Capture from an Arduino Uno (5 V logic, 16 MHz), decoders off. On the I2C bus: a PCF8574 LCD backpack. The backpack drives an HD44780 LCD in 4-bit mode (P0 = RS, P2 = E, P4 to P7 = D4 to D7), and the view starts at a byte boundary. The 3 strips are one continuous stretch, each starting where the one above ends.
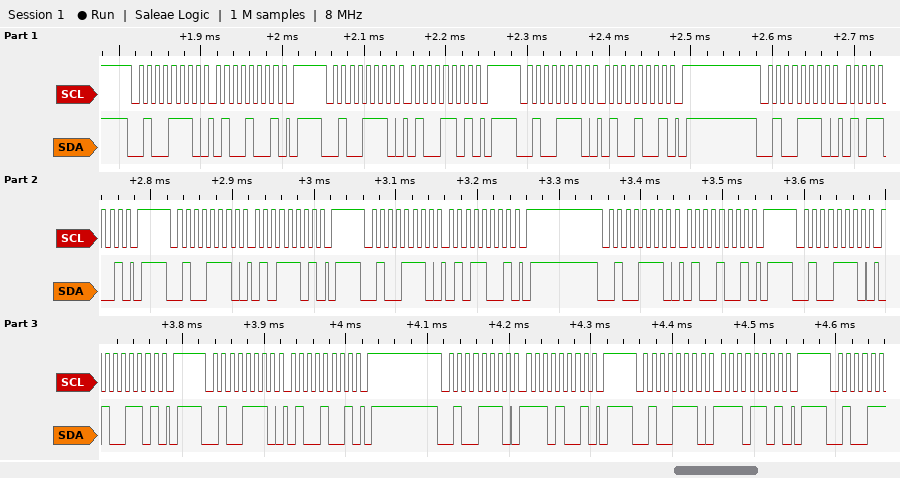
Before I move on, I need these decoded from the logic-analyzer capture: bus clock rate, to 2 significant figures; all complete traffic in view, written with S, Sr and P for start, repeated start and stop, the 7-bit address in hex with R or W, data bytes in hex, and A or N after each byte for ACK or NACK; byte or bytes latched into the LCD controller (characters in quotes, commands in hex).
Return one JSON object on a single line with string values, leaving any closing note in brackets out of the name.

{"bus clock rate, to 2 significant figures": "100 kHz", "all complete traffic in view, written with S, Sr and P for start, repeated start and stop, the 7-bit address in hex with R or W, data bytes in hex, and A or N after each byte for ACK or NACK": "S 27W A 49 A P S 27W A 4D A P S 27W A 49 A P S 27W A 59 A P S 27W A 5D A P S 27W A 59 A P S 27W A 49 A P S 27W A 4D A P S 27W A 49 A P S 27W A E9 A P S 27W A ED A P", "byte or bytes latched into the LCD controller": "'E'"}
